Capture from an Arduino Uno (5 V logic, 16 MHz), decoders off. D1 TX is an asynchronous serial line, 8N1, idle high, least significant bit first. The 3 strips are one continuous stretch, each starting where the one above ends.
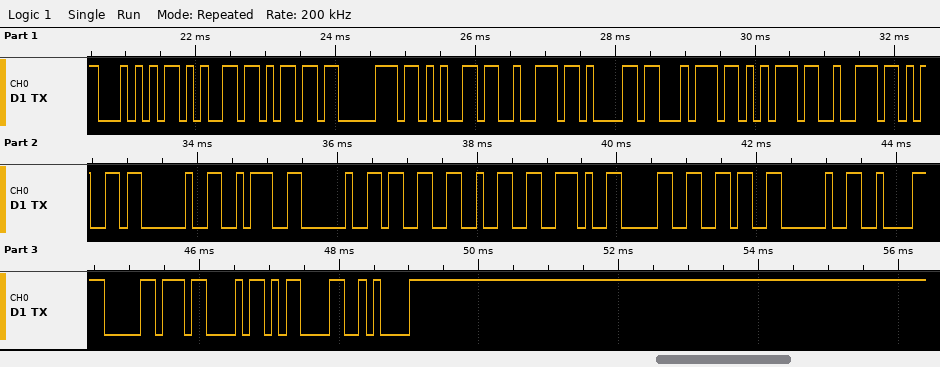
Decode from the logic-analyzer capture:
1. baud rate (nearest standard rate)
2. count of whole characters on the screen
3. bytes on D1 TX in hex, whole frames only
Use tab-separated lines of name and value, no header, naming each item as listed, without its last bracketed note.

baud rate	9600 baud
count of whole characters on the screen	25
bytes on D1 TX in hex, whole frames only	54 65 6D 70 65 72 61 74 75 72 65 20 3A 20 33 32 2E 30 36 20 C2 B0 43 0D 0A
